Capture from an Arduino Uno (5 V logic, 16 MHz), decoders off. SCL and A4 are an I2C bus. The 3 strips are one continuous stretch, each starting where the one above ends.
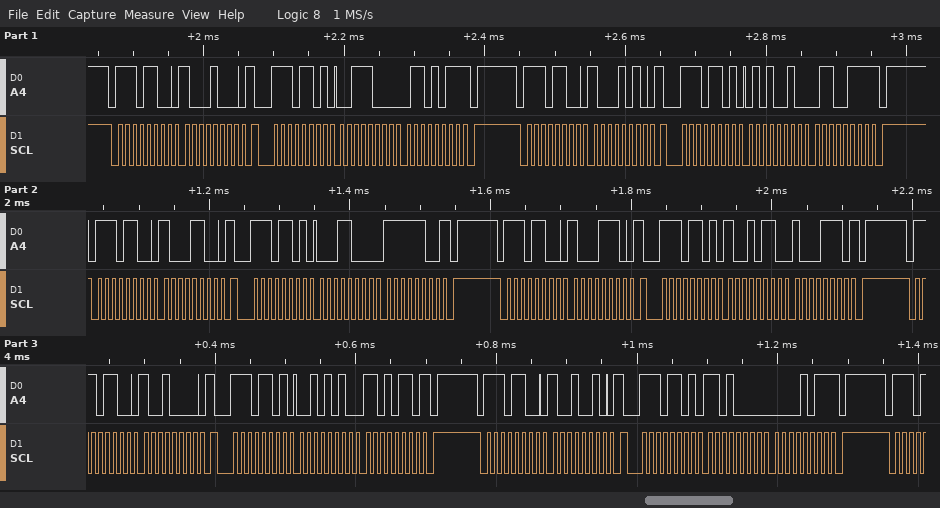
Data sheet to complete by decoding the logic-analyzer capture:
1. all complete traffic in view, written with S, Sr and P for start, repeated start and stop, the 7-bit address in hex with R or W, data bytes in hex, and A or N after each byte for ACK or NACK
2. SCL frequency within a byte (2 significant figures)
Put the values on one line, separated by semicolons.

S 76W A 88 A Sr 76R A 38 A 6B N P S 76W A 8A A Sr 76R A 52 A 67 N P S 76W A 8C A Sr 76R A 18 A FC N P S 76W A 8E A Sr 76R A 96 A 8E N P S 76W A 90 A Sr 76R A 2A A D6 N P S 76W A 92 A Sr 76R A D0 A 0B N P; 100 kHz
